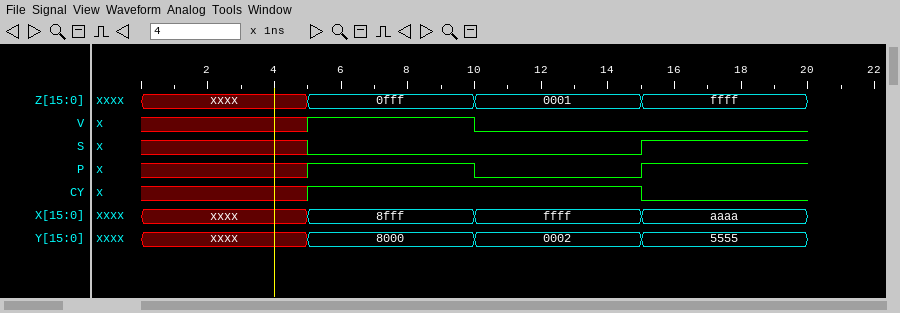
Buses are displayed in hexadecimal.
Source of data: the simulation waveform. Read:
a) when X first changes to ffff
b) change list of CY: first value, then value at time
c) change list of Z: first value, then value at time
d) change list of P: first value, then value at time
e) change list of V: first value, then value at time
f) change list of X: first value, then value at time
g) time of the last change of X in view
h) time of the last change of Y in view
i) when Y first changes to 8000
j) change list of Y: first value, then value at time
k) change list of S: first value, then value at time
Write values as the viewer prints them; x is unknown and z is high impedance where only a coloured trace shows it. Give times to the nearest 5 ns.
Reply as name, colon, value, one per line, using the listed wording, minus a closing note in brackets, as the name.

when X first changes to ffff: 10 ns
change list of CY: first value, then value at time: x, 1 at 5 ns, 0 at 15 ns
change list of Z: first value, then value at time: xxxx, 0fff at 5 ns, 0001 at 10 ns, ffff at 15 ns
change list of P: first value, then value at time: x, 1 at 5 ns, 0 at 10 ns, 1 at 15 ns
change list of V: first value, then value at time: x, 1 at 5 ns, 0 at 10 ns
change list of X: first value, then value at time: xxxx, 8fff at 5 ns, ffff at 10 ns, aaaa at 15 ns
time of the last change of X in view: 15 ns
time of the last change of Y in view: 15 ns
when Y first changes to 8000: 5 ns
change list of Y: first value, then value at time: xxxx, 8000 at 5 ns, 0002 at 10 ns, 5555 at 15 ns
change list of S: first value, then value at time: x, 0 at 5 ns, 1 at 15 ns
